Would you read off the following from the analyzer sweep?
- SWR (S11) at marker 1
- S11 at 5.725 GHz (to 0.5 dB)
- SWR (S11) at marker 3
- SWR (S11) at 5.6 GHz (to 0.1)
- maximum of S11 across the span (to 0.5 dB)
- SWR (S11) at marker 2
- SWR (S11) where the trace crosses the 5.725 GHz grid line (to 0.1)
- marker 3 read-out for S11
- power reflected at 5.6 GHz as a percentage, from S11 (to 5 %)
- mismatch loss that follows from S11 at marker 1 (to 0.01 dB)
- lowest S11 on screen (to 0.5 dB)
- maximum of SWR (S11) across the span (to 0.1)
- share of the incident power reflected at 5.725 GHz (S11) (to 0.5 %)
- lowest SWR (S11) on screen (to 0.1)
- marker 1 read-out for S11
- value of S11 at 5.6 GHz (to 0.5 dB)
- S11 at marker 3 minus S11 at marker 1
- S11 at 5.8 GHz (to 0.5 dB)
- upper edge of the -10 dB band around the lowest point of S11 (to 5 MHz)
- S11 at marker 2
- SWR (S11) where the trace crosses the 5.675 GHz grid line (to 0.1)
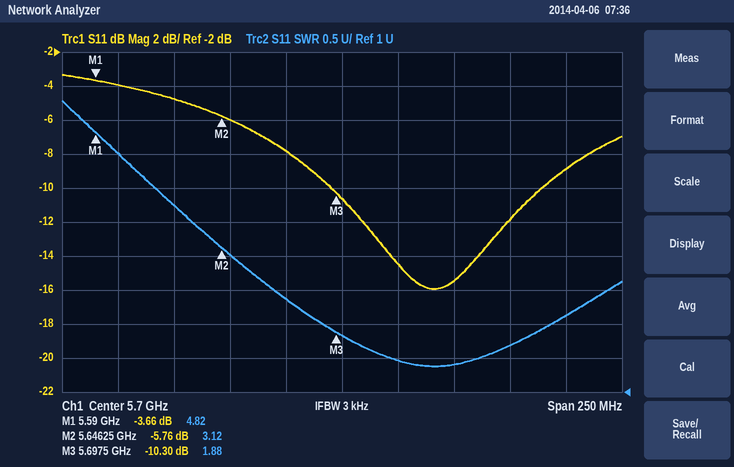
4.82
-14.5 dB
1.88
4.5
-3.5 dB
3.12
1.5
-10.30 dB
40 %
2.45 dB
-16.0 dB
5.3
3.5 %
1.4
-3.66 dB
-4.0 dB
-6.64 dB
-9.0 dB
5.790 GHz
-5.76 dB
2.4
